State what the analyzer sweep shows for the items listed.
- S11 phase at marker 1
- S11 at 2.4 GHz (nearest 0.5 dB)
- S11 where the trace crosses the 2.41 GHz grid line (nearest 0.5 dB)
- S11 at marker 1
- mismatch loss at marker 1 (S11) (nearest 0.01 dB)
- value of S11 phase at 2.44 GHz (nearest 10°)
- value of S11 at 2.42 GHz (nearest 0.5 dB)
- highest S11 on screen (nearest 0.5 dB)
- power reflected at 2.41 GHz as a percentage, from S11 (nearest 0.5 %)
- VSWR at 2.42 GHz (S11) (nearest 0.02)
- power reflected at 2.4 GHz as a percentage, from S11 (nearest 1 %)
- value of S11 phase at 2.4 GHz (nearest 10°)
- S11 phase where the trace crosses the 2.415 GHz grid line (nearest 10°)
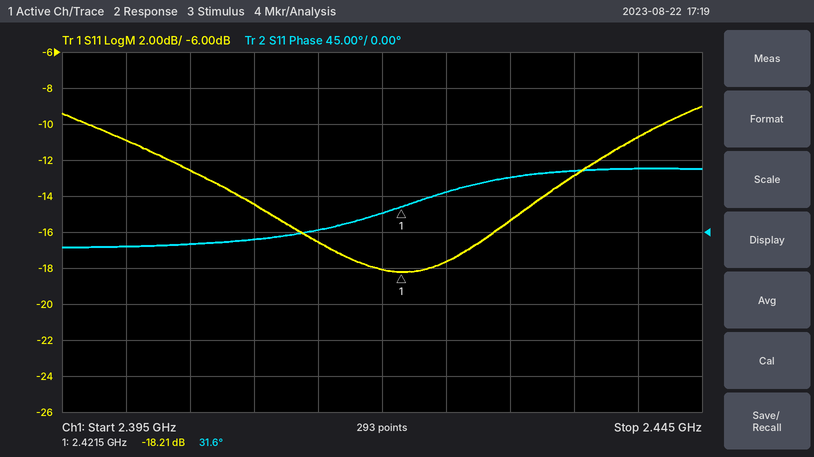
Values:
31.6°
-11.0 dB
-14.5 dB
-18.21 dB
0.07 dB
80°
-18.0 dB
-9.0 dB
3.5 %
1.28
8 %
-20°
0°
